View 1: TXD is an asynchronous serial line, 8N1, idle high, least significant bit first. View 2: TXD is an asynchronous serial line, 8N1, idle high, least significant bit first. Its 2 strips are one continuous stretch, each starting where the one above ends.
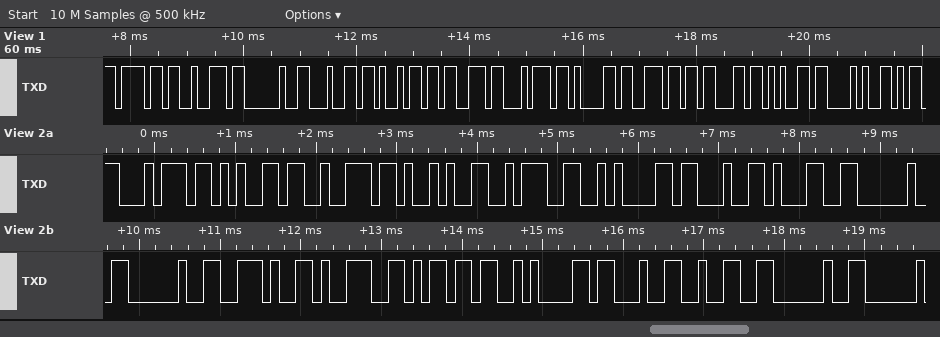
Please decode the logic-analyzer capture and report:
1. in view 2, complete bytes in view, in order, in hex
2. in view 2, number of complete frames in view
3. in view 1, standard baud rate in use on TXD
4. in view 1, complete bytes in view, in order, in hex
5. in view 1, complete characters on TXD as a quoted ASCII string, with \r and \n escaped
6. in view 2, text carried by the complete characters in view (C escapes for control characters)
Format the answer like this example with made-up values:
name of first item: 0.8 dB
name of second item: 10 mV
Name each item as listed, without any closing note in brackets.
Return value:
in view 2, complete bytes in view, in order, in hex: 74 65 72 29 3A 0A 23 31 20 20 2E 39 6D 0A 23 32 20
in view 2, number of complete frames in view: 17
in view 1, standard baud rate in use on TXD: 9600 baud
in view 1, complete bytes in view, in order, in hex: 6F 72 20 64 69 73 74 61 6E 63 65 28
in view 1, complete characters on TXD as a quoted ASCII string, with \r and \n escaped: "or distance("
in view 2, text carried by the complete characters in view: "ter):\n#1  .9m\n#2 "
